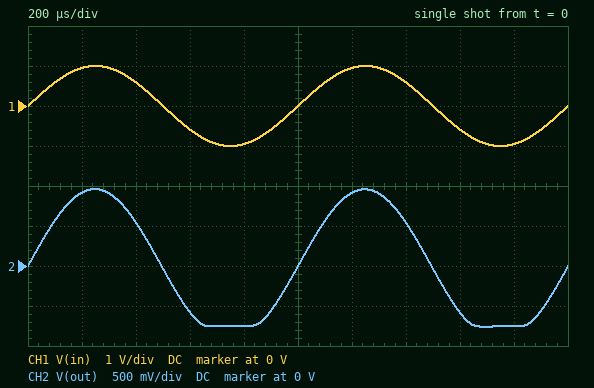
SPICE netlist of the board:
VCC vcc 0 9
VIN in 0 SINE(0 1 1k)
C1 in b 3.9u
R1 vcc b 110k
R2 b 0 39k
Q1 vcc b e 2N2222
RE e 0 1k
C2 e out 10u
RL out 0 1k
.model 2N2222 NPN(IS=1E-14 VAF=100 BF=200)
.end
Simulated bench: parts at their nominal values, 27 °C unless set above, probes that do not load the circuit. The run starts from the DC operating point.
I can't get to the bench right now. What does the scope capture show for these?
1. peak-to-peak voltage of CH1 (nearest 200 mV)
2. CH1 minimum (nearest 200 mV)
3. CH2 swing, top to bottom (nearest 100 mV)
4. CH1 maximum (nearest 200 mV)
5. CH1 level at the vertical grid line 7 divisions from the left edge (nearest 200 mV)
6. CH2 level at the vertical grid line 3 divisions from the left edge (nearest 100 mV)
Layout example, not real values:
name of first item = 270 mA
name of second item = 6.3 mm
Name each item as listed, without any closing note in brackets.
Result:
peak-to-peak voltage of CH1 = 2.0 V
CH1 minimum = -1.0 V
CH2 swing, top to bottom = 1.7 V
CH1 maximum = 1.0 V
CH1 level at the vertical grid line 7 divisions from the left edge = 600 mV
CH2 level at the vertical grid line 3 divisions from the left edge = -600 mV
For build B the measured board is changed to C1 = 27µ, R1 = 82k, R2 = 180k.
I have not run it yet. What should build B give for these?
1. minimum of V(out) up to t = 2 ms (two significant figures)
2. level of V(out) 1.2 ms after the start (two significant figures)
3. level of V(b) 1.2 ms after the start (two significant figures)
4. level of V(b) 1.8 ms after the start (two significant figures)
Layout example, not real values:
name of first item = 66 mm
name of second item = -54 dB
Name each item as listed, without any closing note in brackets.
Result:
minimum of V(out) up to t = 2 ms = -1.0 V
level of V(out) 1.2 ms after the start = 930 mV
level of V(b) 1.2 ms after the start = 6.0 V
level of V(b) 1.8 ms after the start = 4.1 V
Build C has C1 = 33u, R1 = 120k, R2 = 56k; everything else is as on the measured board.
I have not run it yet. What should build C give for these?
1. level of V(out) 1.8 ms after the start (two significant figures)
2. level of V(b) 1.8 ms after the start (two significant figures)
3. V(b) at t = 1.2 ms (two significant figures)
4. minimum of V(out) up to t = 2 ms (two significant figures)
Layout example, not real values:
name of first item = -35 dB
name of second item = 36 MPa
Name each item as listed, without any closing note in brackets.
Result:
level of V(out) 1.8 ms after the start = -890 mV
level of V(b) 1.8 ms after the start = 1.6 V
V(b) at t = 1.2 ms = 3.5 V
minimum of V(out) up to t = 2 ms = -920 mV
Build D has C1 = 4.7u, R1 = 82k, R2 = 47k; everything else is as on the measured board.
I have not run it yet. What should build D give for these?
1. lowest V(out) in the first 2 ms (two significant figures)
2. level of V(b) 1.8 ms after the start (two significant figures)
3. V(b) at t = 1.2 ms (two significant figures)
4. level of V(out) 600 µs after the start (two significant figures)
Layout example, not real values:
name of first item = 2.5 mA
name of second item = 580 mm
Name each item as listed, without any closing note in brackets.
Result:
lowest V(out) in the first 2 ms = -970 mV
level of V(b) 1.8 ms after the start = 2.0 V
V(b) at t = 1.2 ms = 3.9 V
level of V(out) 600 µs after the start = -600 mV
